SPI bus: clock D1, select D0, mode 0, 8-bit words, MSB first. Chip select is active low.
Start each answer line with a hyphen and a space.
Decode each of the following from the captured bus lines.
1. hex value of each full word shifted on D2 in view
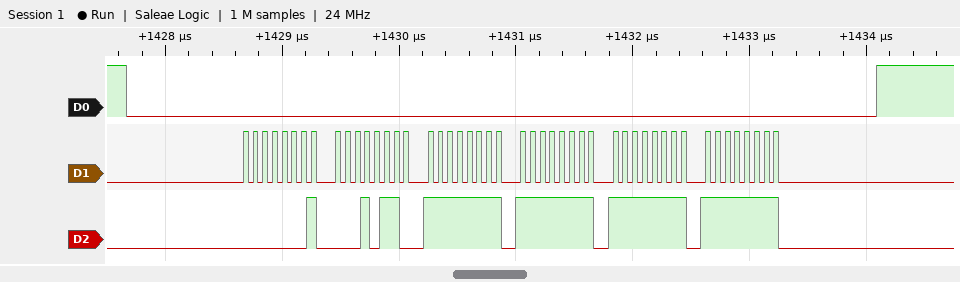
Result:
- 01, 16, FF, FF, FF, FF
